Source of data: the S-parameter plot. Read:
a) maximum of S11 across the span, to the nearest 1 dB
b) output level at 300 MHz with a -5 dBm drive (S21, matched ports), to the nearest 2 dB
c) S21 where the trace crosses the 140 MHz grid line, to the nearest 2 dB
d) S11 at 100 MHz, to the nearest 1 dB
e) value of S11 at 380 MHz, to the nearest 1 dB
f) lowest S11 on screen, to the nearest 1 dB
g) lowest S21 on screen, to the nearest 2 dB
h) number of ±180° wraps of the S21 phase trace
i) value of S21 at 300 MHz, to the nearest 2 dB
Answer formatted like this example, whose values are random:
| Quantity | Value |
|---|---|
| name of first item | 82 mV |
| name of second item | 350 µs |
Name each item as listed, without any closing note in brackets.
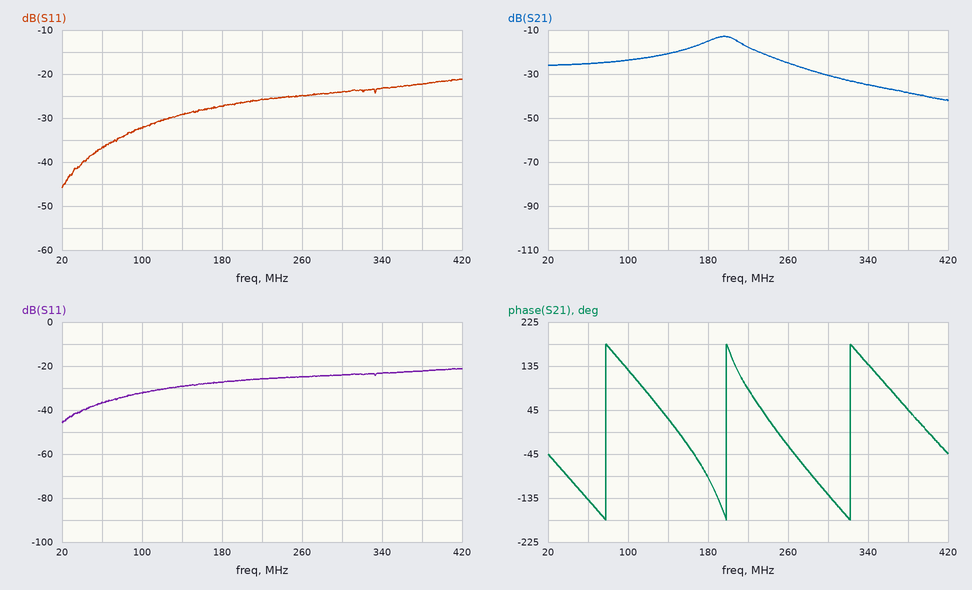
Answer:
| Quantity | Value |
|---|---|
| maximum of S11 across the span, to the nearest 1 dB | -21 dB |
| output level at 300 MHz with a -5 dBm drive (S21, matched ports), to the nearest 2 dB | -36 dBm |
| S21 where the trace crosses the 140 MHz grid line, to the nearest 2 dB | -20 dB |
| S11 at 100 MHz, to the nearest 1 dB | -32 dB |
| value of S11 at 380 MHz, to the nearest 1 dB | -22 dB |
| lowest S11 on screen, to the nearest 1 dB | -46 dB |
| lowest S21 on screen, to the nearest 2 dB | -42 dB |
| number of ±180° wraps of the S21 phase trace | 3 |
| value of S21 at 300 MHz, to the nearest 2 dB | -30 dB |
